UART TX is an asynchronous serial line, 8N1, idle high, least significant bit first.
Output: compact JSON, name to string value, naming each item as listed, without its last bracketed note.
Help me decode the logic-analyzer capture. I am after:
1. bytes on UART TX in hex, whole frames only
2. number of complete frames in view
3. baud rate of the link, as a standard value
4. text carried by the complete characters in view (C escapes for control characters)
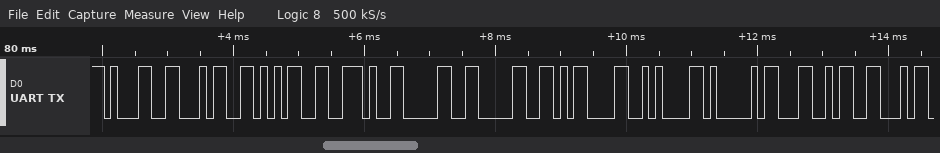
{"bytes on UART TX in hex, whole frames only": "0x31 0x34 0x35 0x2E 0x30 0x30 0x0D 0x0A 0x41 0x4C 0x46", "number of complete frames in view": "11", "baud rate of the link, as a standard value": "9600 baud", "text carried by the complete characters in view": "\"145.00\\r\\nALF\""}
